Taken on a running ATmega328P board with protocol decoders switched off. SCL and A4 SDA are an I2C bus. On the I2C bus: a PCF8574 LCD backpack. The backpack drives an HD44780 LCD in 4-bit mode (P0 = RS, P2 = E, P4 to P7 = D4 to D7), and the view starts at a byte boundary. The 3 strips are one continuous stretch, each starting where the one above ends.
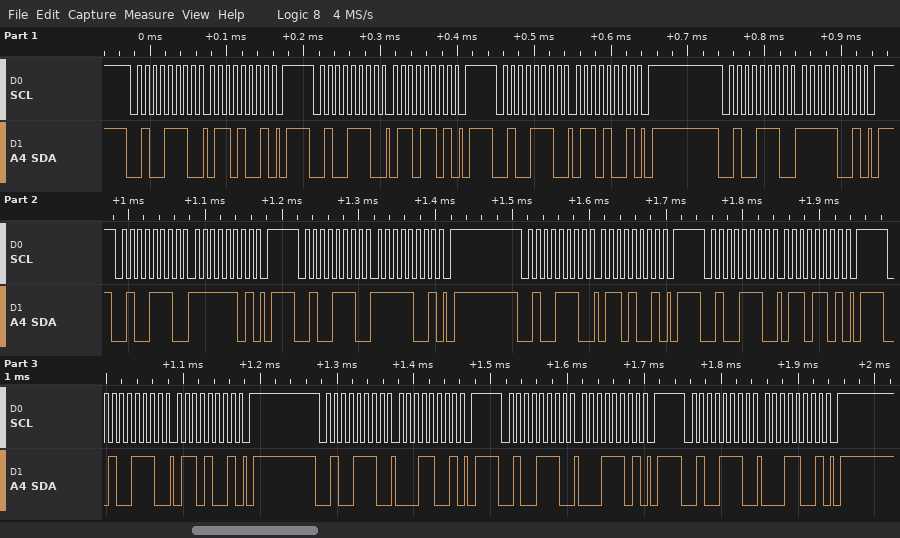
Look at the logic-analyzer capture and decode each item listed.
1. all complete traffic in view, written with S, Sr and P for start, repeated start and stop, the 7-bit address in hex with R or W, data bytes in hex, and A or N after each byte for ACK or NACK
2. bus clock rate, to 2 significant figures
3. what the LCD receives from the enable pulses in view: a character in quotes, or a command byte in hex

S 27W A 69 A P S 27W A 6D A P S 27W A 69 A P S 27W A F9 A P S 27W A FD A P S 27W A F9 A P S 27W A 69 A P S 27W A 6D A P S 27W A 69 A P S 27W A 19 A P S 27W A 1D A P S 27W A 19 A P
100 kHz
'o' 'a'
